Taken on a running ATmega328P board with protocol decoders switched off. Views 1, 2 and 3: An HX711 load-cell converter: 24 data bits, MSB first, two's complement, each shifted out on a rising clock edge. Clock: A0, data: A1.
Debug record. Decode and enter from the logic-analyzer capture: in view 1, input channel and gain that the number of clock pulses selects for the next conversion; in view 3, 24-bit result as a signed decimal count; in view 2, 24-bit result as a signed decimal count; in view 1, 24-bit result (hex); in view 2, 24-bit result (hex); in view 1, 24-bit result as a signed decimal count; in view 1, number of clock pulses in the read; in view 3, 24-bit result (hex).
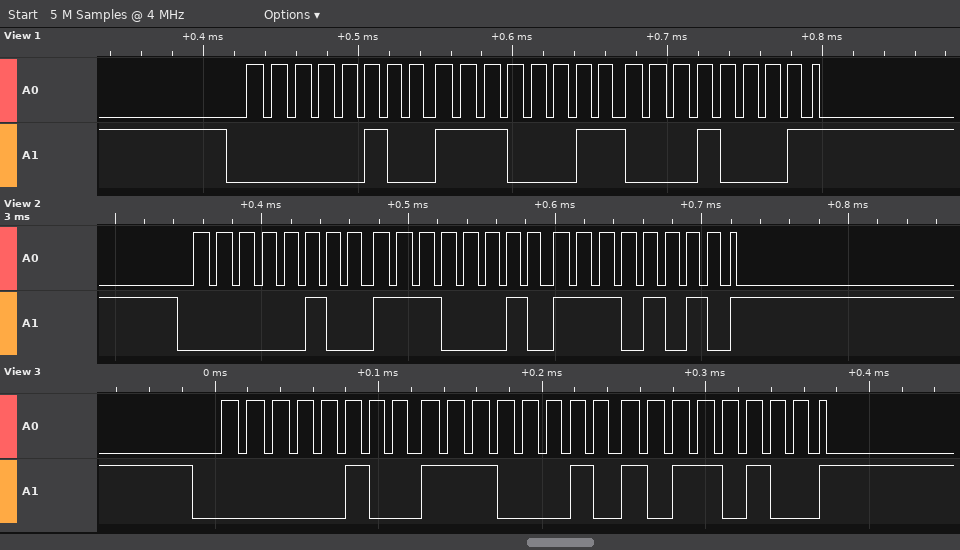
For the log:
channel A, gain 128
320180
320234
0x04E311
0x04E2EA
320273
25
0x04E2B4
